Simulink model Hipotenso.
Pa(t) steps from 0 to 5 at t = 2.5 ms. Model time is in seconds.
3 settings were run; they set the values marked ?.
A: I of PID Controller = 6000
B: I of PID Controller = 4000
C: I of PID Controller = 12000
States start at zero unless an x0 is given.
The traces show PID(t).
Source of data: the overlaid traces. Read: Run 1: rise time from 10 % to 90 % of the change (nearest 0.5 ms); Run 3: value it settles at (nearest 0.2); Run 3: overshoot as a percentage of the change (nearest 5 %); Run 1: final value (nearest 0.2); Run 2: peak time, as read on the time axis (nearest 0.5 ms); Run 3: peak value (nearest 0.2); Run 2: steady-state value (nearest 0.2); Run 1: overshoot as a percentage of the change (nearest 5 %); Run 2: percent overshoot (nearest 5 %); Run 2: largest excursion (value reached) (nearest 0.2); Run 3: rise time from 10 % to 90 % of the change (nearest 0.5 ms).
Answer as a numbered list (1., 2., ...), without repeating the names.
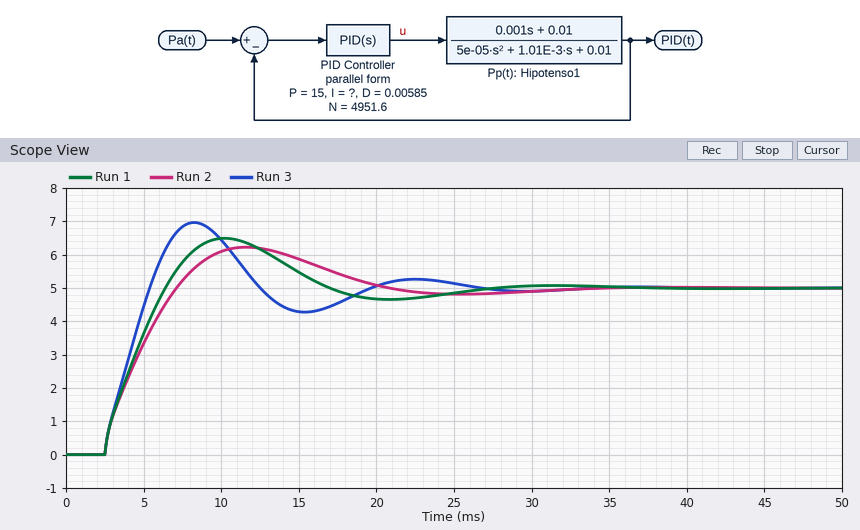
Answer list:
1. 3.0 ms
2. 5.0
3. 40 %
4. 5.0
5. 11.5 ms
6. 7.0
7. 5.0
8. 30 %
9. 25 %
10. 6.2
11. 2.5 ms
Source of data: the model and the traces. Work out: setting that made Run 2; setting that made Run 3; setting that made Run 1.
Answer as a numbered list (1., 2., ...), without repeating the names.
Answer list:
1. B
2. C
3. A
